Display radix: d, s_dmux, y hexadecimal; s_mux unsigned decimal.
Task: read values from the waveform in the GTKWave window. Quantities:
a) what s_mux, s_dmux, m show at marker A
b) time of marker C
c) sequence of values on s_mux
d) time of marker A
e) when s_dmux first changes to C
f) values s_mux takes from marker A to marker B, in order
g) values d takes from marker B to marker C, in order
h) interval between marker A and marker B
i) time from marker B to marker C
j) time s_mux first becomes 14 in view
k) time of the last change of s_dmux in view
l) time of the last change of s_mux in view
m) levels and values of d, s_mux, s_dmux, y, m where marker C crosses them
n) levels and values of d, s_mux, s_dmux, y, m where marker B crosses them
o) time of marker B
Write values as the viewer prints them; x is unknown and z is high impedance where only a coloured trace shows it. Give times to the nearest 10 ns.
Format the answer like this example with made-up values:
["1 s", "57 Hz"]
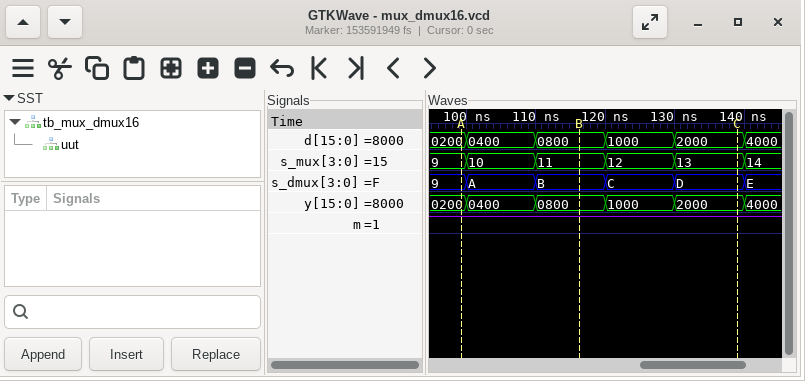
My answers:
["s_mux=9, s_dmux=9, m=1", "140 ns", "9, 10, 11, 12, 13, 14", "100 ns", "120 ns", "9, 10, 11", "0800, 1000, 2000", "20 ns", "20 ns", "140 ns", "140 ns", "140 ns", "d=2000, s_mux=13, s_dmux=D, y=2000, m=1", "d=0800, s_mux=11, s_dmux=B, y=0800, m=1", "120 ns"]
